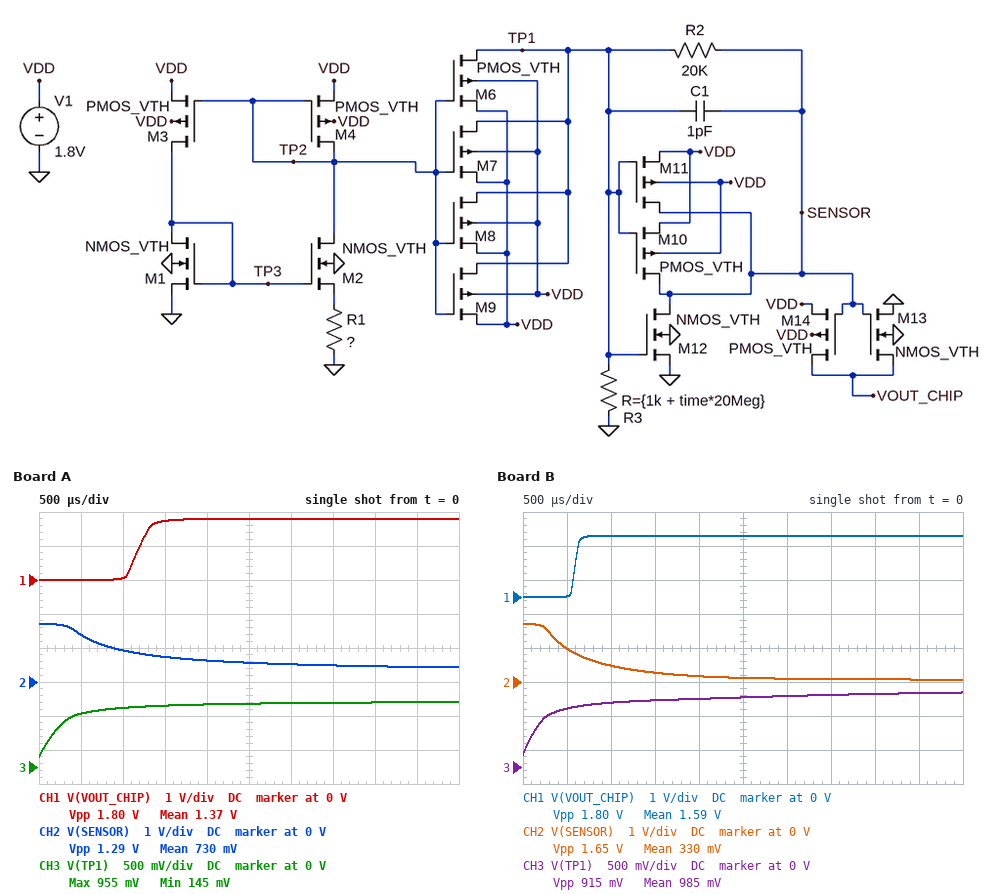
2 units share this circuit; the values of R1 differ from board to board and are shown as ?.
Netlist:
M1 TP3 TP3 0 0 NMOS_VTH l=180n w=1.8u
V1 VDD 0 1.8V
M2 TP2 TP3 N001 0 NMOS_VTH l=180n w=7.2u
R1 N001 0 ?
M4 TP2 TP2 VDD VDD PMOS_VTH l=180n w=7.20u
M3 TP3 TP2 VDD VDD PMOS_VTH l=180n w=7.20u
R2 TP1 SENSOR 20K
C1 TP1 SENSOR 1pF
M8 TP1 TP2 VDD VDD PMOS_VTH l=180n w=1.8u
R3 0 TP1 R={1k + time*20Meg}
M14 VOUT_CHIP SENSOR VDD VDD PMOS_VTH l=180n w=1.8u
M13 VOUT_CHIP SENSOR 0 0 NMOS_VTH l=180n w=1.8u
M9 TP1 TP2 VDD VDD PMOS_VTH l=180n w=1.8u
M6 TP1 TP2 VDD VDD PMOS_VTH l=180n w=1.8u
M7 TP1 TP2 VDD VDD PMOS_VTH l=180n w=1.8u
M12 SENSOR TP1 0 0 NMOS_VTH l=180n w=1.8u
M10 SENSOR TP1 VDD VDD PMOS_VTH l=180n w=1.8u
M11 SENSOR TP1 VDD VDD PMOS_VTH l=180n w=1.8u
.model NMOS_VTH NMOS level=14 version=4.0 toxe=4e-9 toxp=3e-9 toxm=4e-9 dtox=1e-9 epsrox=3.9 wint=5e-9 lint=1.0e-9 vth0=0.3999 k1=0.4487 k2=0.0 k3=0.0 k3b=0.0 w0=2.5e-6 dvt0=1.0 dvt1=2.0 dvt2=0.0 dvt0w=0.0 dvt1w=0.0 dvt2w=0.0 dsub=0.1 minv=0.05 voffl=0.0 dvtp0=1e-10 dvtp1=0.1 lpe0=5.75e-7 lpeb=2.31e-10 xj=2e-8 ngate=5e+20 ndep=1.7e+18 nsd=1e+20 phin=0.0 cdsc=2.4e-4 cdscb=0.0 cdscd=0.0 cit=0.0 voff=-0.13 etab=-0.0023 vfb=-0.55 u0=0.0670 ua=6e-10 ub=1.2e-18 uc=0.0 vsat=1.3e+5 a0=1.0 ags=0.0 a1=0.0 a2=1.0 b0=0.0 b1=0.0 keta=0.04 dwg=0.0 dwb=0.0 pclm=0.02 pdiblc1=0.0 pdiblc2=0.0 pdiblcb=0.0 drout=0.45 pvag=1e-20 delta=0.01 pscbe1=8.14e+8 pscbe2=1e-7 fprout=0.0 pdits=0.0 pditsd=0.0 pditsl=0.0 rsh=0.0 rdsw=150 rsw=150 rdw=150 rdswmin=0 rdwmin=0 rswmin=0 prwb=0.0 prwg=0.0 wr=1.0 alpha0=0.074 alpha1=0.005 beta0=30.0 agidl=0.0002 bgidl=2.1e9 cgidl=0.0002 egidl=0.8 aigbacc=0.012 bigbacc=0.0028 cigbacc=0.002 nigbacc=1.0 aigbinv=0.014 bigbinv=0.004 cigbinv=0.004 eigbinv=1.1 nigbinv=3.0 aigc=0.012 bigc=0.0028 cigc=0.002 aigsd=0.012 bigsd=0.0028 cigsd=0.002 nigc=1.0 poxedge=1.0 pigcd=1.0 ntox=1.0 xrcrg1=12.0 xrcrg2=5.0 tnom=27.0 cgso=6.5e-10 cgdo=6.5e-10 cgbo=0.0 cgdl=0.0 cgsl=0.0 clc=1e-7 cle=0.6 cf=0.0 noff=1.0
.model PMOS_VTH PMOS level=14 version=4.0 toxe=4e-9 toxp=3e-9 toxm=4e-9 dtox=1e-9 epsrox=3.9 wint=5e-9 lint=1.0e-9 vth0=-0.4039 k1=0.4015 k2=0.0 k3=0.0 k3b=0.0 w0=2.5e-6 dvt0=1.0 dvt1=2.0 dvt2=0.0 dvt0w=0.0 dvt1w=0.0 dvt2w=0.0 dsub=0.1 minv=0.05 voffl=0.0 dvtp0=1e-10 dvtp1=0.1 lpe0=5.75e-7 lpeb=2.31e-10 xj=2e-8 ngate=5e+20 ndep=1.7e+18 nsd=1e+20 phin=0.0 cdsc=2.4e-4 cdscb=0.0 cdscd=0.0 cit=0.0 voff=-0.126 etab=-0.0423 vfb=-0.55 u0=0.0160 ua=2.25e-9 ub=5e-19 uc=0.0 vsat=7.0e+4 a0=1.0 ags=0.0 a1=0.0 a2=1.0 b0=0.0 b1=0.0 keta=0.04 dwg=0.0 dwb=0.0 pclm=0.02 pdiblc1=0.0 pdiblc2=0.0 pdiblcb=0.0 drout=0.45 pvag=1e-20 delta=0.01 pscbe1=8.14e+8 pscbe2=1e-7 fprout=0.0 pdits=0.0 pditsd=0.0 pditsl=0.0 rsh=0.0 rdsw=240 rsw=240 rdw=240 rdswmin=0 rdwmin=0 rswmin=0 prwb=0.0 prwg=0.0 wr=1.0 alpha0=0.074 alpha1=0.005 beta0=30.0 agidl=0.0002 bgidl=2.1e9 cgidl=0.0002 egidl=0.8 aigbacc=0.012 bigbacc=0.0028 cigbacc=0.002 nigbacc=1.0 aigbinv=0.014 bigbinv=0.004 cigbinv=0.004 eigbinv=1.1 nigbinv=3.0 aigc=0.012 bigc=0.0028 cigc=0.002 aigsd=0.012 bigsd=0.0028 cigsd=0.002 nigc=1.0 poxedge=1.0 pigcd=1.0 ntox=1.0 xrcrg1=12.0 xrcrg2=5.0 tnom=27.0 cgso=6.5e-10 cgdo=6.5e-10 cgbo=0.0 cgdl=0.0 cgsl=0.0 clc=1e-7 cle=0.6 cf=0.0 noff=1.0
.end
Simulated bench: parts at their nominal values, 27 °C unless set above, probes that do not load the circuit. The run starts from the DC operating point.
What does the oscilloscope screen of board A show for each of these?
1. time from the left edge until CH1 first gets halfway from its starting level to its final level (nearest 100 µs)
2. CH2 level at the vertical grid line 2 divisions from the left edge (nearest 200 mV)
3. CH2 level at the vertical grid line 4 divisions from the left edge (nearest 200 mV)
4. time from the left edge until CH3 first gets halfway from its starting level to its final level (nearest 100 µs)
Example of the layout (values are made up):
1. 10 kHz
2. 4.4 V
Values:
1. 1.2 ms
2. 1.0 V
3. 600 mV
4. 200 µs
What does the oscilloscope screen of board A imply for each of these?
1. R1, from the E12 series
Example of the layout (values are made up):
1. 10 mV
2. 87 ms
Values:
1. 2.2 kΩ
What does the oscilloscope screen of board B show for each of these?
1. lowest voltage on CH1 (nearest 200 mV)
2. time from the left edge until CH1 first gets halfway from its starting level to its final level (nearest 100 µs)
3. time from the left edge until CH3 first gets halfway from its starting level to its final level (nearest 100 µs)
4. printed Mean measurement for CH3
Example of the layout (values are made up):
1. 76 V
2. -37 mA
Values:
1. 0 V
2. 600 µs
3. 200 µs
4. 985 mV
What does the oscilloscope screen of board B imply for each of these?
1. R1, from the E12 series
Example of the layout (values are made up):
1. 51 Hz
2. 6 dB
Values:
1. 1.2 kΩ
